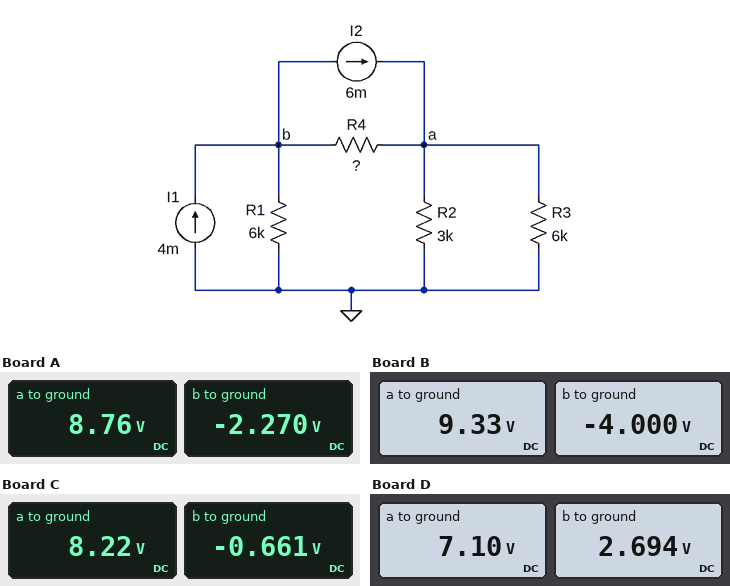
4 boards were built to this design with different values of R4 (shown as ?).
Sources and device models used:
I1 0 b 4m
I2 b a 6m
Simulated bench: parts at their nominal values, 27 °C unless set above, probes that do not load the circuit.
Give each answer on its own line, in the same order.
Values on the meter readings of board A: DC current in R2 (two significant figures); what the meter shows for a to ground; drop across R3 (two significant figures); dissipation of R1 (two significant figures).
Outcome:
2.9 mA
8.76 V
8.8 V
860 µW
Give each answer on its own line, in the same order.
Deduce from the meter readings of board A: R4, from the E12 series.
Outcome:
6.8 kΩ
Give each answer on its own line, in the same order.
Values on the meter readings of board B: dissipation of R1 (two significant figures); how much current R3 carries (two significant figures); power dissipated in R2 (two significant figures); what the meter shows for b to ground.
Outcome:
2.7 mW
1.6 mA
29 mW
-4.000 V
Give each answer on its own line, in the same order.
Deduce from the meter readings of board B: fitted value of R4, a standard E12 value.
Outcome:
10 kΩ
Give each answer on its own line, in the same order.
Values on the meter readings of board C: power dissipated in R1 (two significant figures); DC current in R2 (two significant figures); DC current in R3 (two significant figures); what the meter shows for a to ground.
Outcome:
73 µW
2.7 mA
1.4 mA
8.22 V
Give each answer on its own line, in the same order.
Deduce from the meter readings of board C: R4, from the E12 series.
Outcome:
4.7 kΩ
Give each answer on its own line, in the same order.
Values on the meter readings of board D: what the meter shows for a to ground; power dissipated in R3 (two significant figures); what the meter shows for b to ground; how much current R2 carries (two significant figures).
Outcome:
7.10 V
8.4 mW
2.694 V
2.4 mA
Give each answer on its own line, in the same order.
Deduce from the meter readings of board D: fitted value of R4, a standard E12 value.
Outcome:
1.8 kΩ
